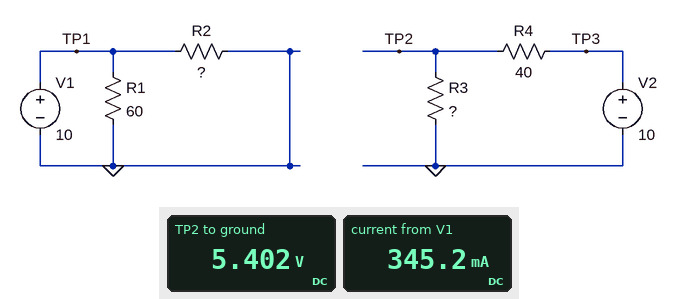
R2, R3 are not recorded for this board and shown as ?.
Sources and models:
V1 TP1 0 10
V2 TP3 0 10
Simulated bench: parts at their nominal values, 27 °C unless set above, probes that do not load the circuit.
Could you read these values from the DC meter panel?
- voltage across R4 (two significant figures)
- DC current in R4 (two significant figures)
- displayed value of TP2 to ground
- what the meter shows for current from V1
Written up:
4.6 V
110 mA
5.402 V
345.2 mA
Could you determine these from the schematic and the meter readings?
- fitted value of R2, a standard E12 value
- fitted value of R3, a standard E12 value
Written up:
56 Ω
47 Ω
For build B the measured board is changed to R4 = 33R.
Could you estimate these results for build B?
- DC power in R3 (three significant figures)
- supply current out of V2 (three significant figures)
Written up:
734 mW
125 mA
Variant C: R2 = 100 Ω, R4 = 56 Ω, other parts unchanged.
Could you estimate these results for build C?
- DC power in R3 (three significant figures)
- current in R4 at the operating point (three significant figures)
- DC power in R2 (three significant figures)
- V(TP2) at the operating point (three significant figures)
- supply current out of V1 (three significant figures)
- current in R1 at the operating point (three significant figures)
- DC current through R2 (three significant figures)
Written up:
443 mW
97.1 mA
1.00 W
4.56 V
267 mA
167 mA
100 mA
